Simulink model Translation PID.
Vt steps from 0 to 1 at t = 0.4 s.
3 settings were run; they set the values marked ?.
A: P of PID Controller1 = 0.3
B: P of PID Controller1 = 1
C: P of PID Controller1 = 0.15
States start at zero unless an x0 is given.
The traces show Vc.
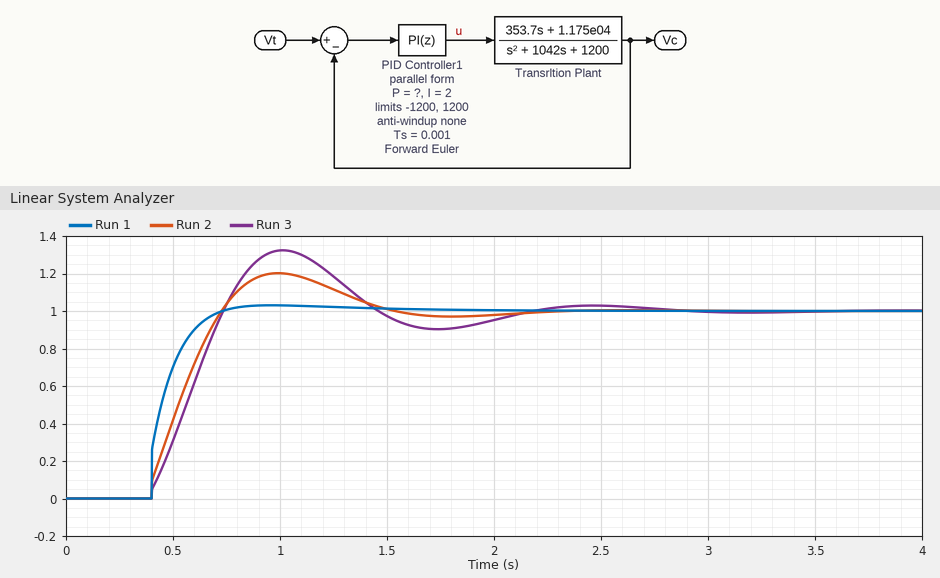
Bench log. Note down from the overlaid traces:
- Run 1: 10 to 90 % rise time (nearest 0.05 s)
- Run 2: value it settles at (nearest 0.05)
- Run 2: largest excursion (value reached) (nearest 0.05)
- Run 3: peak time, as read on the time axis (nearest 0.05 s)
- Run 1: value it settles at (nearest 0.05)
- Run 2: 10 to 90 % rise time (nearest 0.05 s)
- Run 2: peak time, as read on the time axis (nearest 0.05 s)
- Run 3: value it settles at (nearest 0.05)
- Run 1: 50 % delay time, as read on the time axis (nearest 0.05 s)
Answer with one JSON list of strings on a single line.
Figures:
["0.20 s", "1.00", "1.20", "1.00 s", "1.00", "0.25 s", "1.00 s", "1.00", "0.45 s"]
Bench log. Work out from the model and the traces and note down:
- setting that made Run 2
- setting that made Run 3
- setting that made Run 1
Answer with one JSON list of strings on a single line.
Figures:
["A", "C", "B"]
